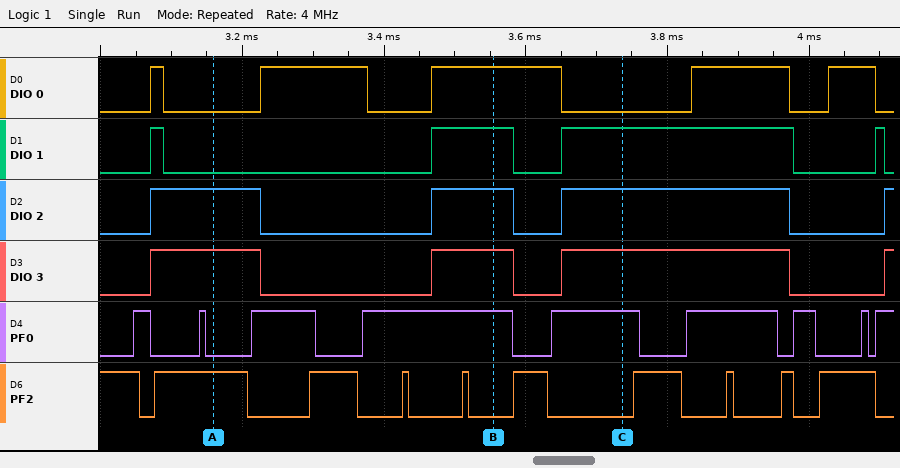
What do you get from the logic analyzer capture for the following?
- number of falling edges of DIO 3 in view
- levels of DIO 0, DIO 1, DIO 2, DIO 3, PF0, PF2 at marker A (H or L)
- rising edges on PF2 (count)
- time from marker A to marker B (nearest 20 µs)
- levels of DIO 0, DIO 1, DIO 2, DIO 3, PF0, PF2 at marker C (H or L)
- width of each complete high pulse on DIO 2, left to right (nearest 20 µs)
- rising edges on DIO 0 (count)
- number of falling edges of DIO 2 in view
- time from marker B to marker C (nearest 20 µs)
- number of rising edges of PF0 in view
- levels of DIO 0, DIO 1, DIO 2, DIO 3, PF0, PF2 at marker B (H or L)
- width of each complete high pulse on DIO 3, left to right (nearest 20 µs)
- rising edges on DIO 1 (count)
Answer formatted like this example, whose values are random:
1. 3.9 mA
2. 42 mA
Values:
1. 3
2. DIO 0=L, DIO 1=L, DIO 2=H, DIO 3=H, PF0=L, PF2=H
3. 9
4. 400 µs
5. DIO 0=L, DIO 1=H, DIO 2=H, DIO 3=H, PF0=H, PF2=L
6. 160 µs, 120 µs, 320 µs
7. 5
8. 3
9. 180 µs
10. 9
11. DIO 0=H, DIO 1=H, DIO 2=H, DIO 3=H, PF0=H, PF2=L
12. 160 µs, 120 µs, 320 µs
13. 4
